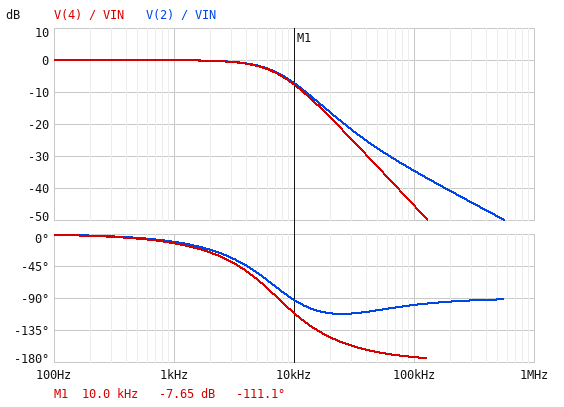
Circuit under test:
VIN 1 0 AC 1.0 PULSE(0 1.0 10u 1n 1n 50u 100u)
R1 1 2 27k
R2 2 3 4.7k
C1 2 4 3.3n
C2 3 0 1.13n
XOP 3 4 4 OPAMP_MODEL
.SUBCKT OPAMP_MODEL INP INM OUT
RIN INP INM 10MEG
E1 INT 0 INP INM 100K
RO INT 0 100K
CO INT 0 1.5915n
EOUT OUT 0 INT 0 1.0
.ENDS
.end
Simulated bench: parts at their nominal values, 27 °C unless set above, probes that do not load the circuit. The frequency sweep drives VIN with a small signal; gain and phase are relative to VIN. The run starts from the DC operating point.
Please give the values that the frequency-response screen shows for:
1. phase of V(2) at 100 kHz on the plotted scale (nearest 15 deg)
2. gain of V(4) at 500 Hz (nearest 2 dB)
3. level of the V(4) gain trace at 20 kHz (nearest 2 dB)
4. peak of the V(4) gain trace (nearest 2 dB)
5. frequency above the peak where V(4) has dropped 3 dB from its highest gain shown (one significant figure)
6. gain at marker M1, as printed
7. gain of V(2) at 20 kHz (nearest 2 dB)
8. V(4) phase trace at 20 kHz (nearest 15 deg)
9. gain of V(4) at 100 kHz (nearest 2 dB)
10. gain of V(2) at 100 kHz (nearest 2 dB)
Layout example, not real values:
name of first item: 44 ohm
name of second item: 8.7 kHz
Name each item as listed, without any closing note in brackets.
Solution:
phase of V(2) at 100 kHz on the plotted scale: -105 deg
gain of V(4) at 500 Hz: 0 dB
level of the V(4) gain trace at 20 kHz: -18 dB
peak of the V(4) gain trace: 0 dB
frequency above the peak where V(4) has dropped 3 dB from its highest gain shown: 6 kHz
gain at marker M1, as printed: -7.65 dB
gain of V(2) at 20 kHz: -16 dB
V(4) phase trace at 20 kHz: -150 deg
gain of V(4) at 100 kHz: -46 dB
gain of V(2) at 100 kHz: -34 dB
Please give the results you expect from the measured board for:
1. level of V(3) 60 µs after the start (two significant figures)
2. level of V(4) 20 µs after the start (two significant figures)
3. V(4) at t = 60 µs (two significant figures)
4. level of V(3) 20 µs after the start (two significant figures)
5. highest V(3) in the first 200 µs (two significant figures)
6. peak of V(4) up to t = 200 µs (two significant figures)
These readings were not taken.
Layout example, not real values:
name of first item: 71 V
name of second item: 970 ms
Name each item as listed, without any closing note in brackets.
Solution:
level of V(3) 60 µs after the start: 750 mV
level of V(4) 20 µs after the start: 82 mV
V(4) at t = 60 µs: 750 mV
level of V(3) 20 µs after the start: 82 mV
highest V(3) in the first 200 µs: 780 mV
peak of V(4) up to t = 200 µs: 780 mV
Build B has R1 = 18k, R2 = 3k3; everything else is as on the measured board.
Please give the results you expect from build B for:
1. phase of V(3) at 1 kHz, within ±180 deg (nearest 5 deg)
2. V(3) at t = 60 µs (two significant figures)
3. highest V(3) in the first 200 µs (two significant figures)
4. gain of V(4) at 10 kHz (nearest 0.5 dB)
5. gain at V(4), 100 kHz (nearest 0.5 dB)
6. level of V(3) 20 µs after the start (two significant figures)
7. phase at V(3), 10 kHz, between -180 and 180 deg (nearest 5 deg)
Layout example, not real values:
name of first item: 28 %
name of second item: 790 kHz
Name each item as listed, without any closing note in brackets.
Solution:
phase of V(3) at 1 kHz, within ±180 deg: -10 deg
V(3) at t = 60 µs: 940 mV
highest V(3) in the first 200 µs: 950 mV
gain of V(4) at 10 kHz: -3.5 dB
gain at V(4), 100 kHz: -39.0 dB
level of V(3) 20 µs after the start: 160 mV
phase at V(3), 10 kHz, between -180 and 180 deg: -85 deg
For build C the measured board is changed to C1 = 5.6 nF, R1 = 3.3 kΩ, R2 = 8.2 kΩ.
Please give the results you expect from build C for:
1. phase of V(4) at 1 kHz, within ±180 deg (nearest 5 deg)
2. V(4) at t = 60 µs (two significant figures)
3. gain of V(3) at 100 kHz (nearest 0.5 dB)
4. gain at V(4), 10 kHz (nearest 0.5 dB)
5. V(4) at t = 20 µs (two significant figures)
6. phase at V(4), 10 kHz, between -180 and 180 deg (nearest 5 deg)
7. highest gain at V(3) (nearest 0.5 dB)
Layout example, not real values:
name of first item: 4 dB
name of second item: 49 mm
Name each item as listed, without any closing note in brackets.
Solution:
phase of V(4) at 1 kHz, within ±180 deg: -5 deg
V(4) at t = 60 µs: 1.2 V
gain of V(3) at 100 kHz: -36.5 dB
gain at V(4), 10 kHz: 1.0 dB
V(4) at t = 20 µs: 220 mV
phase at V(4), 10 kHz, between -180 and 180 deg: -70 deg
highest gain at V(3): 1.5 dB
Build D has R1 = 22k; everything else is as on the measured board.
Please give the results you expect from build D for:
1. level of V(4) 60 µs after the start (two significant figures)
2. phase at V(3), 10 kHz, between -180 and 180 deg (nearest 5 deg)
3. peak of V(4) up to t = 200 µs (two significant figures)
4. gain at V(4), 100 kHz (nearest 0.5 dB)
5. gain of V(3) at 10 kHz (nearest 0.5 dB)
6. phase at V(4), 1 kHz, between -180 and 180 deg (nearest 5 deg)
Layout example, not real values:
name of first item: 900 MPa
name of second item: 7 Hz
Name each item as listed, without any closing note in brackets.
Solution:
level of V(4) 60 µs after the start: 840 mV
phase at V(3), 10 kHz, between -180 and 180 deg: -105 deg
peak of V(4) up to t = 200 µs: 860 mV
gain at V(4), 100 kHz: -43.5 dB
gain of V(3) at 10 kHz: -6.0 dB
phase at V(4), 1 kHz, between -180 and 180 deg: -10 deg
